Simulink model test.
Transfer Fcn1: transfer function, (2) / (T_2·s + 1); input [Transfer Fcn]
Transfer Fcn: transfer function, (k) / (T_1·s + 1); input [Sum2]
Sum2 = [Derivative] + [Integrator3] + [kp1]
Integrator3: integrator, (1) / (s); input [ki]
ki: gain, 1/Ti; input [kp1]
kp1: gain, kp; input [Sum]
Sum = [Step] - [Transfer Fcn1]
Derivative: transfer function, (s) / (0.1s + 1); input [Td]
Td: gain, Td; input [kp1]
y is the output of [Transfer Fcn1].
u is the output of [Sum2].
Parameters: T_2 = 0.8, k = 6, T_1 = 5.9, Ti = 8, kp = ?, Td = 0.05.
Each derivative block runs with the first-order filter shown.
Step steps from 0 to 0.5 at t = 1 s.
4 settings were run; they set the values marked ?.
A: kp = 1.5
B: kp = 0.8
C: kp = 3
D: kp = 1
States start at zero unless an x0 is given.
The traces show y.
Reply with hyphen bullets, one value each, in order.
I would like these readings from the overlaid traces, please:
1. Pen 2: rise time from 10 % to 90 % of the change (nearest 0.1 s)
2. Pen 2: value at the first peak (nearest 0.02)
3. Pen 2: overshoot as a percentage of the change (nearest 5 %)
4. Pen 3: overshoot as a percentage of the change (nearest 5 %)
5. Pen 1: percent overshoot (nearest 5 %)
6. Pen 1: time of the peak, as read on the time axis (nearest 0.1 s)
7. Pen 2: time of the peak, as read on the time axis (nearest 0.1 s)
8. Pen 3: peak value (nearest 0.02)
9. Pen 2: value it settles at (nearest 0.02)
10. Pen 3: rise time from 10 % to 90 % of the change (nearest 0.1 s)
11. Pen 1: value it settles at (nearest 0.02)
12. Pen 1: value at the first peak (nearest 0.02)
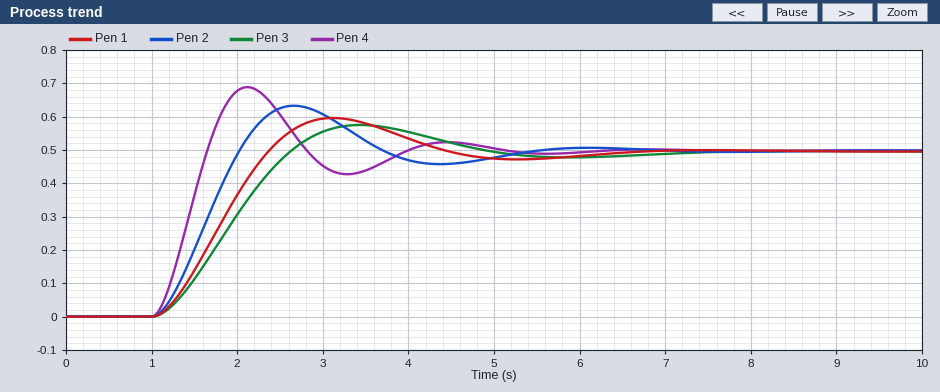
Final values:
- 0.7 s
- 0.64
- 25 %
- 15 %
- 20 %
- 3.1 s
- 2.7 s
- 0.58
- 0.50
- 1.1 s
- 0.50
- 0.60
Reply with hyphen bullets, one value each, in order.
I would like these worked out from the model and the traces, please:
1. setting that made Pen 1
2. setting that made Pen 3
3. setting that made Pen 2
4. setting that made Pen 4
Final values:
- D
- B
- A
- C
